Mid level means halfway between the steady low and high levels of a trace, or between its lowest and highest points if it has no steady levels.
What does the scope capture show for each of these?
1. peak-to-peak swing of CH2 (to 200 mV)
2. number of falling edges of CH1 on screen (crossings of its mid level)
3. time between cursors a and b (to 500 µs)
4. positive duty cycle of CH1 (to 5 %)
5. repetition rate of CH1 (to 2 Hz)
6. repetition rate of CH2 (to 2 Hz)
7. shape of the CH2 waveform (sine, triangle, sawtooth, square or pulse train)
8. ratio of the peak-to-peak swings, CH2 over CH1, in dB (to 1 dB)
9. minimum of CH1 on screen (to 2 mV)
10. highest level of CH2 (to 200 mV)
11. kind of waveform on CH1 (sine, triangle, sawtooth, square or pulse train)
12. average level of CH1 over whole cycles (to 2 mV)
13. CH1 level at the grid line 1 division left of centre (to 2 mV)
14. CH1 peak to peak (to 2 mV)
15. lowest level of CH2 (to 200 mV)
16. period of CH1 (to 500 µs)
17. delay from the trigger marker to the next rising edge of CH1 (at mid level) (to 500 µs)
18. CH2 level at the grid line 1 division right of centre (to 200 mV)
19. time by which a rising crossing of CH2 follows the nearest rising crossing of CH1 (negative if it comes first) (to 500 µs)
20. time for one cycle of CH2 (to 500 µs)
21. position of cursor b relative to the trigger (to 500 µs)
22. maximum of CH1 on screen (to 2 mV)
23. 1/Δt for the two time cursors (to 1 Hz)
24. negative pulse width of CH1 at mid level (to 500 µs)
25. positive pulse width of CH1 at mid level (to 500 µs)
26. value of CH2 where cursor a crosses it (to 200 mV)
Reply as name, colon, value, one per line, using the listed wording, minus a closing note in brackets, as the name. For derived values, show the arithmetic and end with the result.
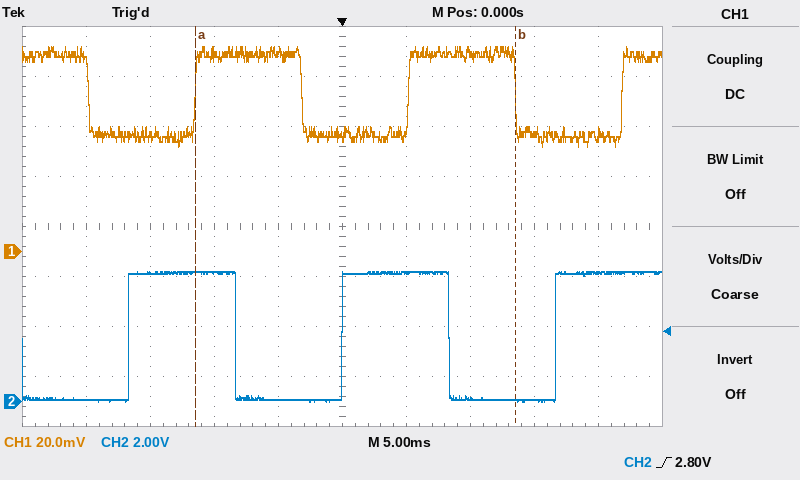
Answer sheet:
peak-to-peak swing of CH2: 5.2 V − (0.0 V) = 5.2 V
number of falling edges of CH1 on screen: 3
time between cursors a and b: 25.0 ms
positive duty cycle of CH1: 8.5 ms / 16.5 ms ≈ 51.5 %, so 50 % to the nearest 5 %
repetition rate of CH1: 1 / 16.5 ms ≈ 60.6 Hz, so 60 Hz to the nearest 2 Hz
repetition rate of CH2: 1 / 16.5 ms ≈ 60.6 Hz, so 60 Hz to the nearest 2 Hz
shape of the CH2 waveform: square
ratio of the peak-to-peak swings, CH2 over CH1, in dB: 20 log10(5.2 V / 40 mV) ≈ 42 dB
minimum of CH1 on screen: 42 mV
highest level of CH2: 5.2 V
kind of waveform on CH1: square
average level of CH1 over whole cycles: 42 mV + 0.5 × (82 mV − (42 mV)) ≈ 62 mV
CH1 level at the grid line 1 division left of centre: 80 mV
CH1 peak to peak: 82 mV − (42 mV) = 40 mV
lowest level of CH2: 0.0 V
period of CH1: 16.5 ms
delay from the trigger marker to the next rising edge of CH1 (at mid level): 5.0 ms
CH2 level at the grid line 1 division right of centre: 5.2 V
time by which a rising crossing of CH2 follows the nearest rising crossing of CH1 (negative if it comes first): -5.0 ms
time for one cycle of CH2: 16.5 ms
position of cursor b relative to the trigger: +13.5 ms
maximum of CH1 on screen: 82 mV
1/Δt for the two time cursors: 1 / 25.0 ms ≈ 40 Hz
negative pulse width of CH1 at mid level: 8.5 ms
positive pulse width of CH1 at mid level: 8.5 ms
value of CH2 where cursor a crosses it: 5.2 V
